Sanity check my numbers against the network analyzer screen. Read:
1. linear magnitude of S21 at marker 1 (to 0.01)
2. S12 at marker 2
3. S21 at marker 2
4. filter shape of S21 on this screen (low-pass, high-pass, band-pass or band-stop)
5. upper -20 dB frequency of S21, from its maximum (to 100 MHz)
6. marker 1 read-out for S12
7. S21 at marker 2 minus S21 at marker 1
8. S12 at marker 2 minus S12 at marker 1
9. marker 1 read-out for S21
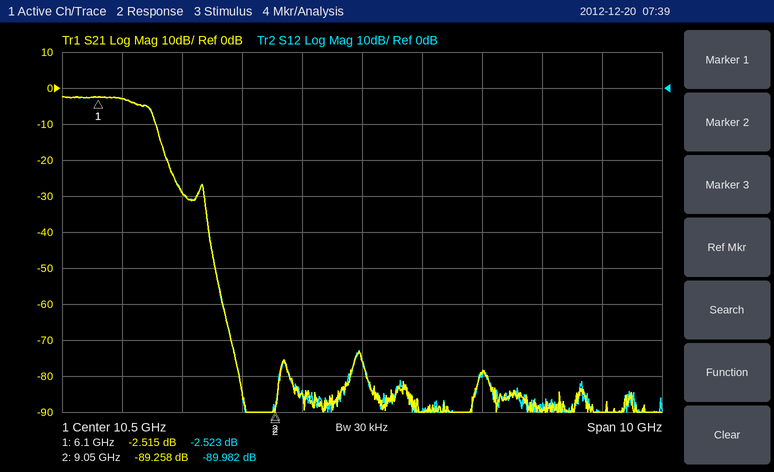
0.75
-89.982 dB
-89.258 dB
low-pass
7.3 GHz
-2.523 dB
-86.743 dB
-87.459 dB
-2.515 dB
